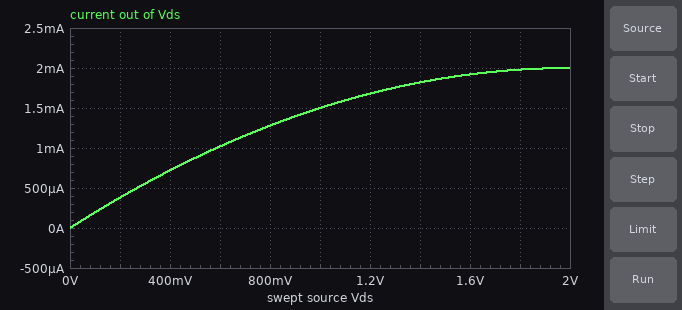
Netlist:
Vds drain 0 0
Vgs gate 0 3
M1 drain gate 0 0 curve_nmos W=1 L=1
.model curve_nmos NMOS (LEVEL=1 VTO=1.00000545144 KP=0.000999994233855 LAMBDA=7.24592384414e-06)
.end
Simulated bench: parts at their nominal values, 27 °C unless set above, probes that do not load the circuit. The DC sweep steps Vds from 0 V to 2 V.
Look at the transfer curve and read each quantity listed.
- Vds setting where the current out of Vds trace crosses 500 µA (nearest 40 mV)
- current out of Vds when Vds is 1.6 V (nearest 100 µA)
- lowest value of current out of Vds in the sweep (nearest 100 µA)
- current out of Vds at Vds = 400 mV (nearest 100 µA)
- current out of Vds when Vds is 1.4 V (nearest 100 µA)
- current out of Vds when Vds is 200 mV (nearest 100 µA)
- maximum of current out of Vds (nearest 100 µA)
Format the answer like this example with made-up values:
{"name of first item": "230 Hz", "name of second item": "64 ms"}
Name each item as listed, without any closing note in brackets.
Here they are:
{"Vds setting where the current out of Vds trace crosses 500 µA": "280 mV", "current out of Vds when Vds is 1.6 V": "1.9 mA", "lowest value of current out of Vds in the sweep": "0 A", "current out of Vds at Vds = 400 mV": "700 µA", "current out of Vds when Vds is 1.4 V": "1.8 mA", "current out of Vds when Vds is 200 mV": "400 µA", "maximum of current out of Vds": "2.0 mA"}
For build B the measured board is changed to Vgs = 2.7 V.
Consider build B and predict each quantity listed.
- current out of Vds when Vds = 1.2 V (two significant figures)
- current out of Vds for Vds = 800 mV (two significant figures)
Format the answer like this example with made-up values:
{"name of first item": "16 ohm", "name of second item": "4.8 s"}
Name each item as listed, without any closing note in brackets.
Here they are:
{"current out of Vds when Vds = 1.2 V": "1.3 mA", "current out of Vds for Vds = 800 mV": "1.0 mA"}
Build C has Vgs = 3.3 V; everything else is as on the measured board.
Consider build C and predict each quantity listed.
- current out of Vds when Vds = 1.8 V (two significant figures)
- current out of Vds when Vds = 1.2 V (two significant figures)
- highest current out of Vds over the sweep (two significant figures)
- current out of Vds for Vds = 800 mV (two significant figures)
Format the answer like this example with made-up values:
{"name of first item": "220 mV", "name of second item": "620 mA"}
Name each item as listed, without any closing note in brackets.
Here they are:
{"current out of Vds when Vds = 1.8 V": "2.5 mA", "current out of Vds when Vds = 1.2 V": "2.0 mA", "highest current out of Vds over the sweep": "2.6 mA", "current out of Vds for Vds = 800 mV": "1.5 mA"}
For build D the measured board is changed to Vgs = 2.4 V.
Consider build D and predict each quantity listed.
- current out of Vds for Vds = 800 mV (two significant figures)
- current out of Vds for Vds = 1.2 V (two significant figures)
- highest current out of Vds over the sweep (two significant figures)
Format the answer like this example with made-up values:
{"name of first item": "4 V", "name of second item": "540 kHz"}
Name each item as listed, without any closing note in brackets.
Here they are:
{"current out of Vds for Vds = 800 mV": "800 µA", "current out of Vds for Vds = 1.2 V": "960 µA", "highest current out of Vds over the sweep": "980 µA"}
